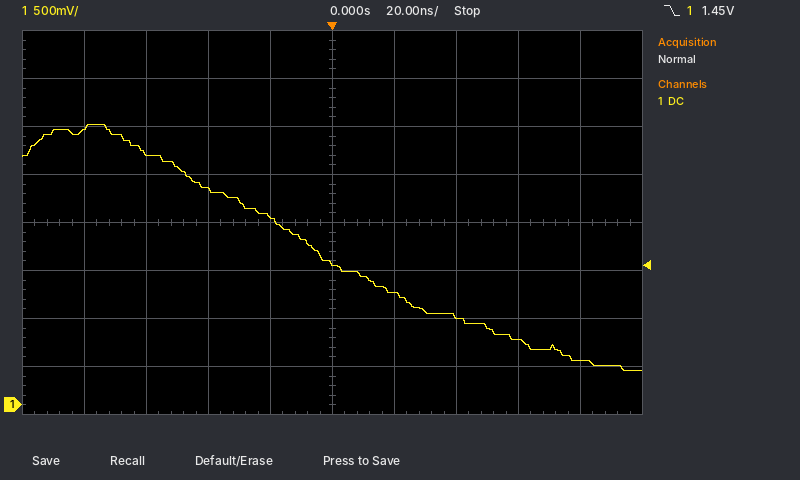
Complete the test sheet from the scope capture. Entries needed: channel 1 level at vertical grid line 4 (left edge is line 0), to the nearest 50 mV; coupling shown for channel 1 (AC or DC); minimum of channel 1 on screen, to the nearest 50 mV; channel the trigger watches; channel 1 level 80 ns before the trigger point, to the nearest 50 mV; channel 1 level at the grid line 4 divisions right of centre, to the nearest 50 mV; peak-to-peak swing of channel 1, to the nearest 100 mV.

1.95 V
DC
350 mV
channel 1
2.90 V
450 mV
2.60 V
